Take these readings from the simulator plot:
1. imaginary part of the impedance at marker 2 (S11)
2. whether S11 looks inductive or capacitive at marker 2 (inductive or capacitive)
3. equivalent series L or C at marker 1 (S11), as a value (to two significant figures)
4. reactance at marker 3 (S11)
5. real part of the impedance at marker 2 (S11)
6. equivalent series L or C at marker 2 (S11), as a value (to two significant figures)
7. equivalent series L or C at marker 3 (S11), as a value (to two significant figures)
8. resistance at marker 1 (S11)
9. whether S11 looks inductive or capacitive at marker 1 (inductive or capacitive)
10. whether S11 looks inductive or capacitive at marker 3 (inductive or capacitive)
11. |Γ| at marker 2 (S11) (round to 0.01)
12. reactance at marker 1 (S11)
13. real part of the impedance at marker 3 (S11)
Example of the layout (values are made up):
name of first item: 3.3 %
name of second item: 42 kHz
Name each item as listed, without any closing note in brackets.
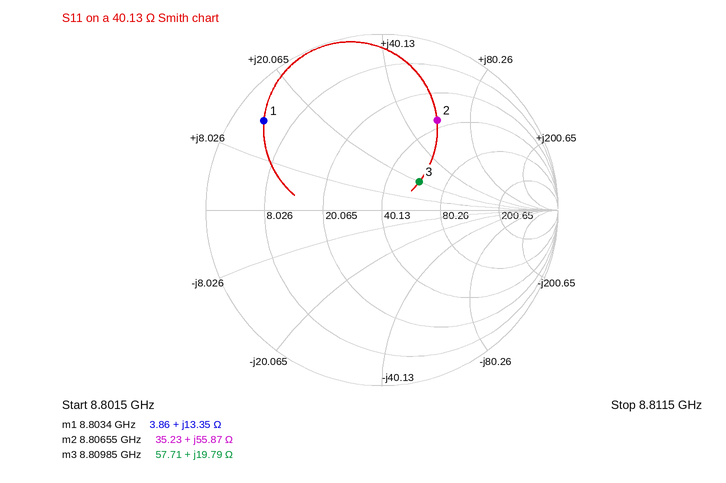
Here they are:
imaginary part of the impedance at marker 2: +55.87 Ω
whether S11 looks inductive or capacitive at marker 2: inductive
equivalent series L or C at marker 1 (S11), as a value: 240 pH
reactance at marker 3: +19.79 Ω
real part of the impedance at marker 2: 35.23 Ω
equivalent series L or C at marker 2 (S11), as a value: 1.0 nH
equivalent series L or C at marker 3 (S11), as a value: 360 pH
resistance at marker 1: 3.86 Ω
whether S11 looks inductive or capacitive at marker 1: inductive
whether S11 looks inductive or capacitive at marker 3: inductive
|Γ| at marker 2 (S11): 0.60
reactance at marker 1: +13.35 Ω
real part of the impedance at marker 3: 57.71 Ω
